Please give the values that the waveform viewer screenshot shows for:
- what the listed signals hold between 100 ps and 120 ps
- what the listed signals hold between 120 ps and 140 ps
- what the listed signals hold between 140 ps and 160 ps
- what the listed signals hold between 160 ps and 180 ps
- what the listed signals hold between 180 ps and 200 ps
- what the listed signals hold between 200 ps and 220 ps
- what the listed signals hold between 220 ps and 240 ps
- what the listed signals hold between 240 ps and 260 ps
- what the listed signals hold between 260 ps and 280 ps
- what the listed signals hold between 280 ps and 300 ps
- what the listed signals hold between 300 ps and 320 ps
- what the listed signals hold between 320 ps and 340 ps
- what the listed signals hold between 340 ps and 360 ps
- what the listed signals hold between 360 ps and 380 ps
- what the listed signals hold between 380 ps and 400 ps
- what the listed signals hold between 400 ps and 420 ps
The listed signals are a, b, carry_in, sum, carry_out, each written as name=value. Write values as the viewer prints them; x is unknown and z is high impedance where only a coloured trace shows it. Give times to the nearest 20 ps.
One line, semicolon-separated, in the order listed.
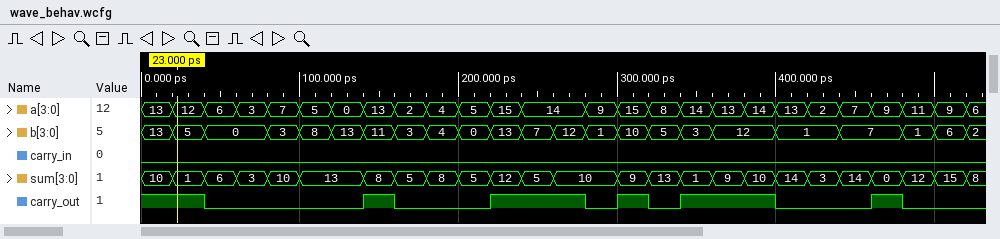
a=5, b=8, carry_in=0, sum=13, carry_out=0; a=0, b=13, carry_in=0, sum=13, carry_out=0; a=13, b=11, carry_in=0, sum=8, carry_out=1; a=2, b=3, carry_in=0, sum=5, carry_out=0; a=4, b=4, carry_in=0, sum=8, carry_out=0; a=5, b=0, carry_in=0, sum=5, carry_out=0; a=15, b=13, carry_in=0, sum=12, carry_out=1; a=14, b=7, carry_in=0, sum=5, carry_out=1; a=14, b=12, carry_in=0, sum=10, carry_out=1; a=9, b=1, carry_in=0, sum=10, carry_out=0; a=15, b=10, carry_in=0, sum=9, carry_out=1; a=8, b=5, carry_in=0, sum=13, carry_out=0; a=14, b=3, carry_in=0, sum=1, carry_out=1; a=13, b=12, carry_in=0, sum=9, carry_out=1; a=14, b=12, carry_in=0, sum=10, carry_out=1; a=13, b=1, carry_in=0, sum=14, carry_out=0
